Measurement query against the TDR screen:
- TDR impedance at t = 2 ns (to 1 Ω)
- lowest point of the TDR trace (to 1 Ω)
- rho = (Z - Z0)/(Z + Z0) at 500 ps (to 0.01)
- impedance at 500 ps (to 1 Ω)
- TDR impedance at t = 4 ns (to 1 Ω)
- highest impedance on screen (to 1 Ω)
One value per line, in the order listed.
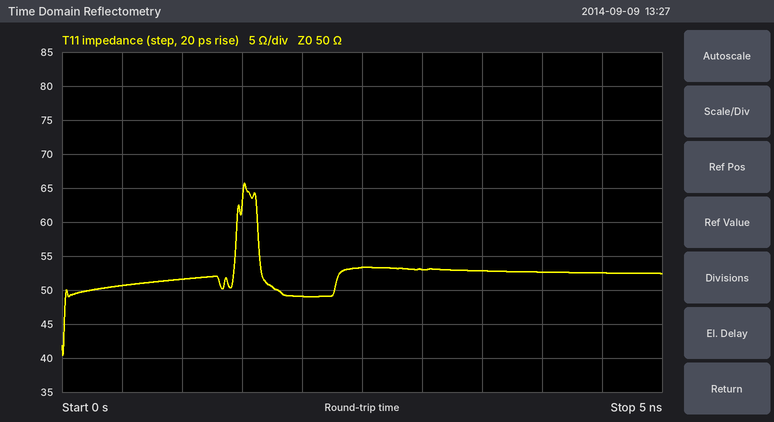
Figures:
49 Ω
40 Ω
+0.01
51 Ω
53 Ω
66 Ω
